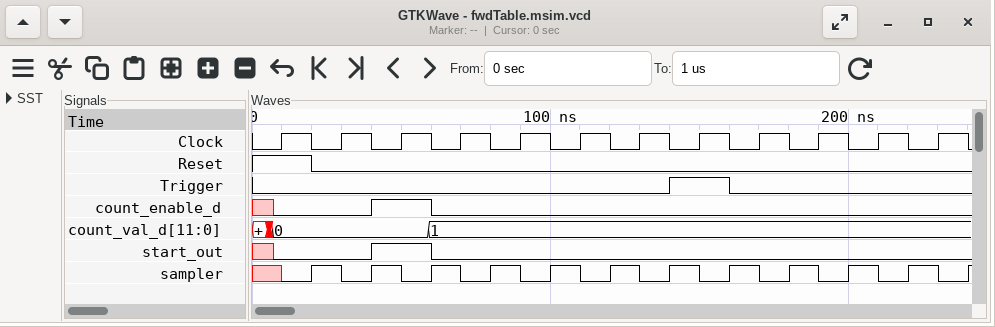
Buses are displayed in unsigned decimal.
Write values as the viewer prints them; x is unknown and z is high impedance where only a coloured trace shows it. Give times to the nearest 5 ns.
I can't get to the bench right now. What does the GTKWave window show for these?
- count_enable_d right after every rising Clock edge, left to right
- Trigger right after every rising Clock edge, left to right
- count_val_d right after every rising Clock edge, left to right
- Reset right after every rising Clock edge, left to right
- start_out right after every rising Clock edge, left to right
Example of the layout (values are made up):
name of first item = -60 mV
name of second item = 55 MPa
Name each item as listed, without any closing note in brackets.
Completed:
count_enable_d right after every rising Clock edge, left to right = 0 0 1 0 0 0 0 0 0 0 0 0
Trigger right after every rising Clock edge, left to right = 0 0 0 0 0 0 0 1 0 0 0 0
count_val_d right after every rising Clock edge, left to right = 0, 0, 0, 1, 1, 1, 1, 1, 1, 1, 1, 1
Reset right after every rising Clock edge, left to right = 1 0 0 0 0 0 0 0 0 0 0 0
start_out right after every rising Clock edge, left to right = 0 0 1 0 0 0 0 0 0 0 0 0
